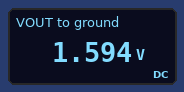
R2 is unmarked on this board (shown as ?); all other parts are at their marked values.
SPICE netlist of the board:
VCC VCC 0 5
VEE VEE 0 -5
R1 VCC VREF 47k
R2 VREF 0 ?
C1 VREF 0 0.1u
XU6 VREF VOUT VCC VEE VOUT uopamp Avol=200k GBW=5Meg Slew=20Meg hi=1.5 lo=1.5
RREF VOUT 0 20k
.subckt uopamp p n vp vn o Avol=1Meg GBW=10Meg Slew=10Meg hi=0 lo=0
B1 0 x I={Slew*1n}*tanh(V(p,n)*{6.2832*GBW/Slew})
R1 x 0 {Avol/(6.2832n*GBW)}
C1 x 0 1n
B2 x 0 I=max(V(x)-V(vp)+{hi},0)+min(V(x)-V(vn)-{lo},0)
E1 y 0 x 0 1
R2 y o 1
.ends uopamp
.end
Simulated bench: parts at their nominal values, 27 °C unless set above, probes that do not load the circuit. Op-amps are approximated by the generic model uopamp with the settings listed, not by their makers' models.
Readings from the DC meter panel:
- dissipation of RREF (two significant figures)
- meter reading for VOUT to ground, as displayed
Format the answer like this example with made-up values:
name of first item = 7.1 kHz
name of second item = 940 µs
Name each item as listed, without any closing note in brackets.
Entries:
dissipation of RREF = 130 µW
meter reading for VOUT to ground, as displayed = 1.594 V
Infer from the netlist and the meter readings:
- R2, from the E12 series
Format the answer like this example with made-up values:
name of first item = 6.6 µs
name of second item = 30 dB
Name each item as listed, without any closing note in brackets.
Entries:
R2, from the E12 series = 22 kΩ
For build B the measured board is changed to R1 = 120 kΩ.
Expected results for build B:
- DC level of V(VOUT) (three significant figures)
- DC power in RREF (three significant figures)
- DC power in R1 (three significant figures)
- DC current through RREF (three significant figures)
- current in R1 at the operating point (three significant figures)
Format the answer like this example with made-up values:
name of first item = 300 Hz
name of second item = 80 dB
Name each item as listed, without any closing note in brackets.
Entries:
DC level of V(VOUT) = 775 mV
DC power in RREF = 30.0 µW
DC power in R1 = 149 µW
DC current through RREF = 38.7 µA
current in R1 at the operating point = 35.2 µA
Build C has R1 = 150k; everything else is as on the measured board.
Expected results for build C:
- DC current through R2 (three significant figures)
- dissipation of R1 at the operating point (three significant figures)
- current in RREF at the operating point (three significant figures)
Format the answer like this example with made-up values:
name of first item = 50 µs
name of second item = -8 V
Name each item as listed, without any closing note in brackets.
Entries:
DC current through R2 = 29.1 µA
dissipation of R1 at the operating point = 127 µW
current in RREF at the operating point = 32.0 µA
